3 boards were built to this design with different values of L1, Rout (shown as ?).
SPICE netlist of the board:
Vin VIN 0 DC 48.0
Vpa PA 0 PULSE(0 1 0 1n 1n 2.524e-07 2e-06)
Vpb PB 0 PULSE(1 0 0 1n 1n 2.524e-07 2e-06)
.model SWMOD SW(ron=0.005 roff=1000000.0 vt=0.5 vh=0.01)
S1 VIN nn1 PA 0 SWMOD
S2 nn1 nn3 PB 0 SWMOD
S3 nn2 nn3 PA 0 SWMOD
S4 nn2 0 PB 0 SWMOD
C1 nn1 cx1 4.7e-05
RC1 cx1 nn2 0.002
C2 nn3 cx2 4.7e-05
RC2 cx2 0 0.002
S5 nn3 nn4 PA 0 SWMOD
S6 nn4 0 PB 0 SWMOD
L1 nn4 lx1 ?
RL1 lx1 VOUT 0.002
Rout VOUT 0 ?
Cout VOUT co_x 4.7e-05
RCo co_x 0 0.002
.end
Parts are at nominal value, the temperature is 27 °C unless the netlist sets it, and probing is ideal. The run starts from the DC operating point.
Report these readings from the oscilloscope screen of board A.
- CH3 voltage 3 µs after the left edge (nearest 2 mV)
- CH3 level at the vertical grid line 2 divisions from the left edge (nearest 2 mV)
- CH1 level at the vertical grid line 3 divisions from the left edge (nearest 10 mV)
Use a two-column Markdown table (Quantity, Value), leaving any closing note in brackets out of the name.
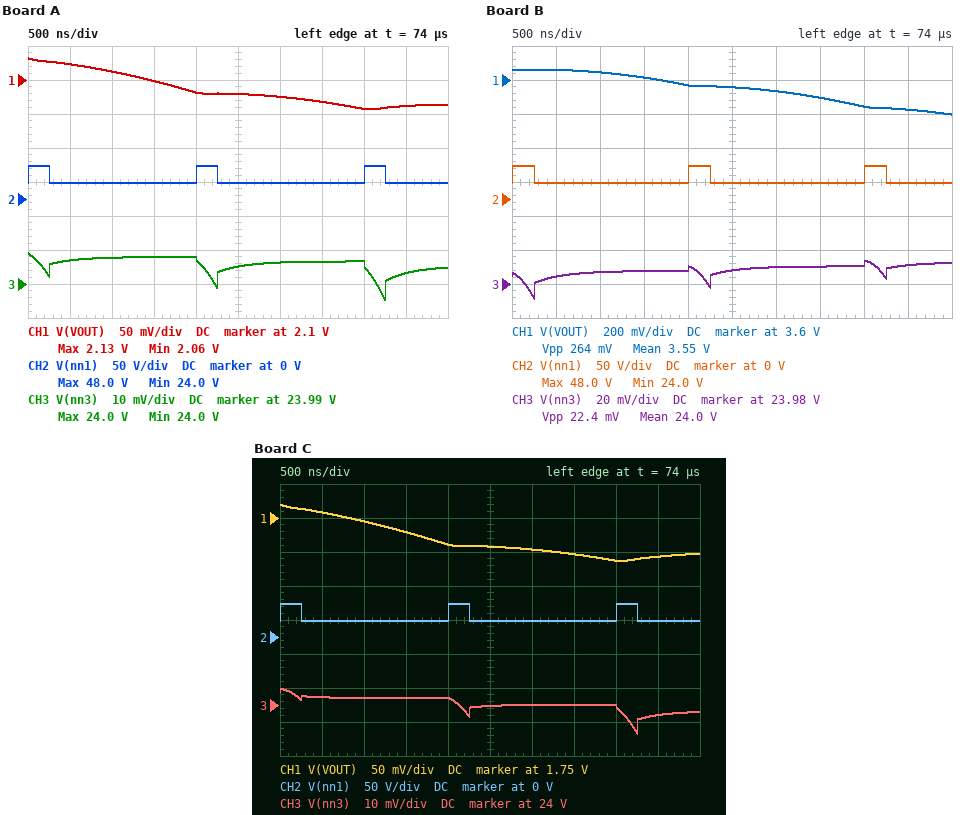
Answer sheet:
| Quantity | Value |
|---|---|
| CH3 voltage 3 µs after the left edge | 23.996 V |
| CH3 level at the vertical grid line 2 divisions from the left edge | 23.998 V |
| CH1 level at the vertical grid line 3 divisions from the left edge | 2.10 V |
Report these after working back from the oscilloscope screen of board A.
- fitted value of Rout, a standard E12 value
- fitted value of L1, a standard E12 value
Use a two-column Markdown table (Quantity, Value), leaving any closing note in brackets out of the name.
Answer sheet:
| Quantity | Value |
|---|---|
| fitted value of Rout, a standard E12 value | 0.82 Ω |
| fitted value of L1, a standard E12 value | 3.3 µH |
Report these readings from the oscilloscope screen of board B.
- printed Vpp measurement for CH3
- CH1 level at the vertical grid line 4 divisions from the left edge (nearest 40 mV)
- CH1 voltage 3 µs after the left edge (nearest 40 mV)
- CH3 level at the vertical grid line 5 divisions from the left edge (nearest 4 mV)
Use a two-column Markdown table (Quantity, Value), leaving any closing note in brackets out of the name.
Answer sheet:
| Quantity | Value |
|---|---|
| printed Vpp measurement for CH3 | 22.4 mV |
| CH1 level at the vertical grid line 4 divisions from the left edge | 3.56 V |
| CH1 voltage 3 µs after the left edge | 3.52 V |
| CH3 level at the vertical grid line 5 divisions from the left edge | 23.988 V |
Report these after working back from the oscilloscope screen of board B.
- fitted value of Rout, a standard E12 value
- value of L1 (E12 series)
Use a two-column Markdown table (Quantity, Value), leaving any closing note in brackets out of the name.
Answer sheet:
| Quantity | Value |
|---|---|
| fitted value of Rout, a standard E12 value | 0.68 Ω |
| value of L1 | 1.2 µH |
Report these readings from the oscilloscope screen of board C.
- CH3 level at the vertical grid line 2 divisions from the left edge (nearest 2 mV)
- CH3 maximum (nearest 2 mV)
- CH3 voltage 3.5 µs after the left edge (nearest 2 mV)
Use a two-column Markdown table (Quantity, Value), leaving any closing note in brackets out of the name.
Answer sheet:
| Quantity | Value |
|---|---|
| CH3 level at the vertical grid line 2 divisions from the left edge | 24.002 V |
| CH3 maximum | 24.004 V |
| CH3 voltage 3.5 µs after the left edge | 24.000 V |
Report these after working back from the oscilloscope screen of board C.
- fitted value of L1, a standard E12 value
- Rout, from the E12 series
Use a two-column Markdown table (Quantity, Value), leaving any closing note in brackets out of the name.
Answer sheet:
| Quantity | Value |
|---|---|
| fitted value of L1, a standard E12 value | 3.3 µH |
| Rout, from the E12 series | 1.2 Ω |
